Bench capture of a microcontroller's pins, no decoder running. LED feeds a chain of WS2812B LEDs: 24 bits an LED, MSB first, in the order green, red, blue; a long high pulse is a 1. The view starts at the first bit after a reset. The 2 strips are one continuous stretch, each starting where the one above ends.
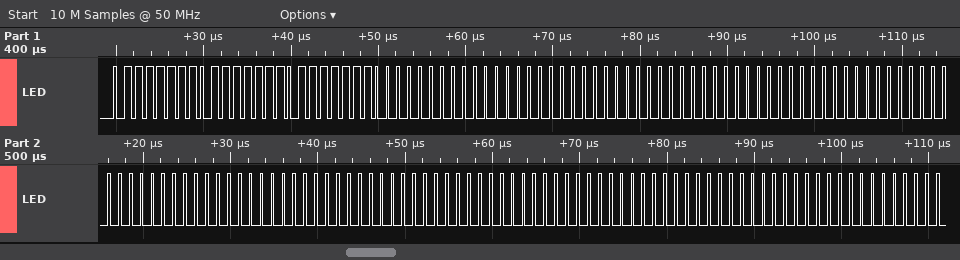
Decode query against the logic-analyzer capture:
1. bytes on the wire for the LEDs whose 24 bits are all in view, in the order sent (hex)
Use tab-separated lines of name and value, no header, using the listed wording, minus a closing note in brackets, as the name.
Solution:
bytes on the wire for the LEDs whose 24 bits are all in view, in the order sent	7F 7F 7F 00 00 00 00 00 00 00 00 00 00 00 00 00 00 00
